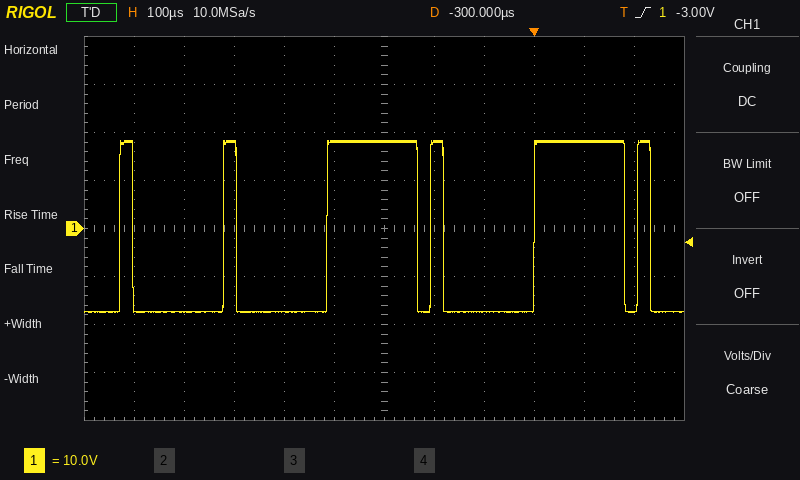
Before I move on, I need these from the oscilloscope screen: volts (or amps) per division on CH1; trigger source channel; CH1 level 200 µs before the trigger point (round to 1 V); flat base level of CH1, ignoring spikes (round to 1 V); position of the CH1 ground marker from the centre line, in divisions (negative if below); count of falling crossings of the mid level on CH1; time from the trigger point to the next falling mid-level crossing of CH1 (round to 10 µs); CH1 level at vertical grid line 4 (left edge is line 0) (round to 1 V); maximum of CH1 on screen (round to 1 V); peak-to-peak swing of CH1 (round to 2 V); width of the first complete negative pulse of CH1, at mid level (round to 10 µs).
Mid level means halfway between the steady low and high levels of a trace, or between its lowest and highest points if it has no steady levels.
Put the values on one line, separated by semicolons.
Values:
10 V; CH1; 18 V; -17 V; 0.0 div; 6; 180 µs; -17 V; 18 V; 36 V; 180 µs
